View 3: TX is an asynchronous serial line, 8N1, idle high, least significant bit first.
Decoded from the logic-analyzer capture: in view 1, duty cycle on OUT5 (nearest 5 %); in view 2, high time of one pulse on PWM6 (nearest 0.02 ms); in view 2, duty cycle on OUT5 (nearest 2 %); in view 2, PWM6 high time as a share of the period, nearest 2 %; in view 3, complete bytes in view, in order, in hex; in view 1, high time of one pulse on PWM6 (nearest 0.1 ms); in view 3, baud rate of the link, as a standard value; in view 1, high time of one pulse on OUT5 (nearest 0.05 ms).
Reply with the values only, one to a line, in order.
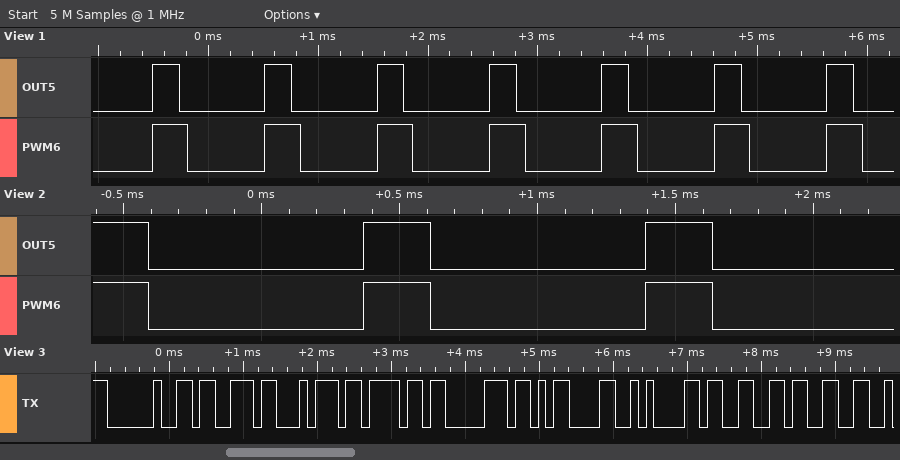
25 %
0.24 ms
24 %
24 %
20 73 74 6F 70 0D 0A 33 33
0.3 ms
9600 baud
0.25 ms
